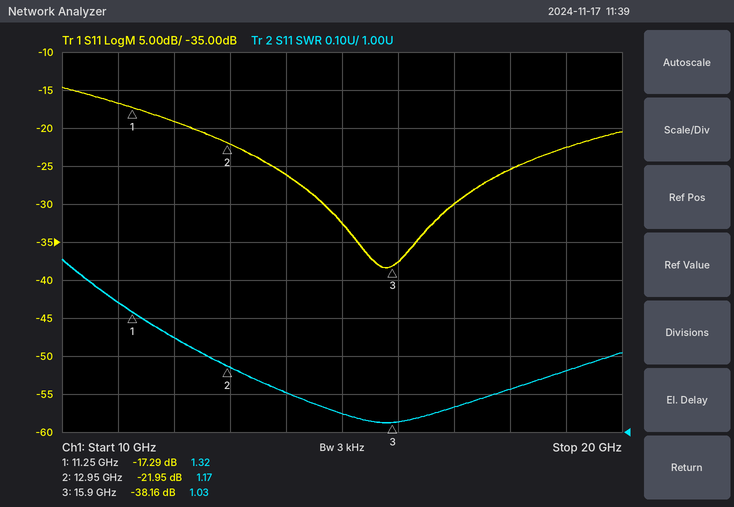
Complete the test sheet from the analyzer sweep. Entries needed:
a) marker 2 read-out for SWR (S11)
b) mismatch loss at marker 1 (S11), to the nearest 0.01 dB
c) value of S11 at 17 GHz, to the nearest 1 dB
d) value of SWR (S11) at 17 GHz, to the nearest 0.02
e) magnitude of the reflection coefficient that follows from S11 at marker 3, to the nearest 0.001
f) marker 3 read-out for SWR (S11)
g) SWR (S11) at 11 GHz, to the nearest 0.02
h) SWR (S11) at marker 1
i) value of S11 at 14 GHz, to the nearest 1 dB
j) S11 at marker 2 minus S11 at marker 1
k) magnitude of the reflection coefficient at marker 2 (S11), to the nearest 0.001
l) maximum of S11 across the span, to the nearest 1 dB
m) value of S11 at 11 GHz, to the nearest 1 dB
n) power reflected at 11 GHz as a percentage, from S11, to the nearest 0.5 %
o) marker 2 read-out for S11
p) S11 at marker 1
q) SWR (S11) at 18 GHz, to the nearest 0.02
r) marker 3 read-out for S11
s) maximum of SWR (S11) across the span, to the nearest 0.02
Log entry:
1.17
0.08 dB
-30 dB
1.06
0.012
1.03
1.34
1.32
-26 dB
-4.66 dB
0.080
-15 dB
-17 dB
2.0 %
-21.95 dB
-17.29 dB
1.12
-38.16 dB
1.46
